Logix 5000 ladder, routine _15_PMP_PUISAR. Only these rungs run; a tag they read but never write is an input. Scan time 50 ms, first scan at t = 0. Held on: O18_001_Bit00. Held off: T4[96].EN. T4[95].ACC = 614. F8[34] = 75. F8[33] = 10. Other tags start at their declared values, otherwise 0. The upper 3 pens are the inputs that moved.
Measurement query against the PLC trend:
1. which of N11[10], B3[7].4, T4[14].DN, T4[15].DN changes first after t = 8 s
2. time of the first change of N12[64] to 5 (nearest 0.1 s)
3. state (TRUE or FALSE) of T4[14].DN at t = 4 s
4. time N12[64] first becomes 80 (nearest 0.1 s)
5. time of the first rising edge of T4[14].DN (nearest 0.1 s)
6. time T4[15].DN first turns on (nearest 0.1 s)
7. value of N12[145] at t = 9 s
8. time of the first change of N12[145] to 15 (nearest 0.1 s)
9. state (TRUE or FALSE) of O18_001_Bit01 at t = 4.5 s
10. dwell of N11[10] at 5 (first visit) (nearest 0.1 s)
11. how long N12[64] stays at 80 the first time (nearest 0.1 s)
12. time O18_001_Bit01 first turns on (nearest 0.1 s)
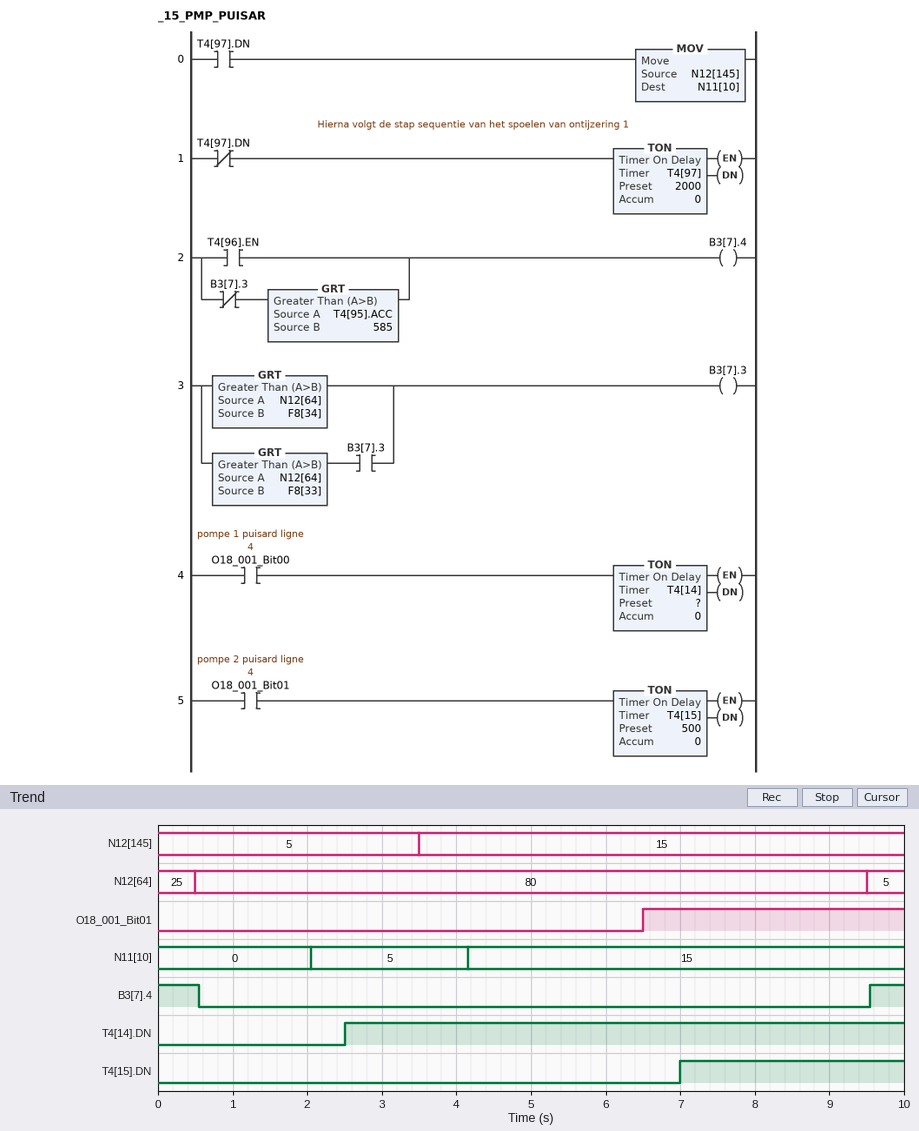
B3[7].4
9.5 s
TRUE
0.5 s
2.5 s
7.0 s
15
3.5 s
FALSE
2.1 s
9.0 s
6.5 s
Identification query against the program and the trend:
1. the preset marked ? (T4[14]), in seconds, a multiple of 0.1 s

2.5 s
